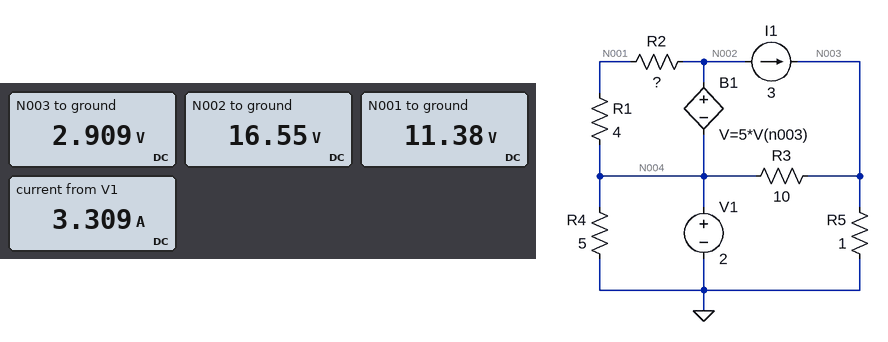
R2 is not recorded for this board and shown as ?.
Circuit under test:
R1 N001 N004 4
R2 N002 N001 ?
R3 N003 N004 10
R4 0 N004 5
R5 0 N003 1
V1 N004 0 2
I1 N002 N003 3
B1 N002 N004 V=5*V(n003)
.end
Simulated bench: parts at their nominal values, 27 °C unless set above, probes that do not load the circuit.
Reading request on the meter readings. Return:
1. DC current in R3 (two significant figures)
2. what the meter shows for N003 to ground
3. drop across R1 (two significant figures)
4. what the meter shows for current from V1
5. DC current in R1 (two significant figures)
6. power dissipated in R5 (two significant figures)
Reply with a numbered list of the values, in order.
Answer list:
1. 91 mA
2. 2.909 V
3. 9.4 V
4. 3.309 A
5. 2.3 A
6. 8.5 W
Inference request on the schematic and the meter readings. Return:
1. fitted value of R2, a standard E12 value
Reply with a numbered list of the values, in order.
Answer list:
1. 2.2 Ω
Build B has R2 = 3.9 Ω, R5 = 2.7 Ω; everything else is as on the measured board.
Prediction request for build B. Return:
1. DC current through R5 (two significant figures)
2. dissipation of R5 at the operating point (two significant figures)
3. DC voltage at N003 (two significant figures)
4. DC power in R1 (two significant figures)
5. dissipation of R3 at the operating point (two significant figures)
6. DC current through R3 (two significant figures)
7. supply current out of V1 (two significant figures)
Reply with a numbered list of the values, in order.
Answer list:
1. 2.5 A
2. 17 W
3. 6.8 V
4. 74 W
5. 2.3 W
6. 480 mA
7. 2.9 A
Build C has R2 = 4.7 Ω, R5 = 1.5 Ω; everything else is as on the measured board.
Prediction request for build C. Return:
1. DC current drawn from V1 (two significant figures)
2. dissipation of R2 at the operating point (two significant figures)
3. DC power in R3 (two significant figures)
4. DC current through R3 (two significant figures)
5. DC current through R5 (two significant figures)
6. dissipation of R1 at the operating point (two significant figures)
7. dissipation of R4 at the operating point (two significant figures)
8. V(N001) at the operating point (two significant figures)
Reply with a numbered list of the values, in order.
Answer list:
1. 3.2 A
2. 27 W
3. 470 mW
4. 220 mA
5. 2.8 A
6. 23 W
7. 800 mW
8. 12 V
